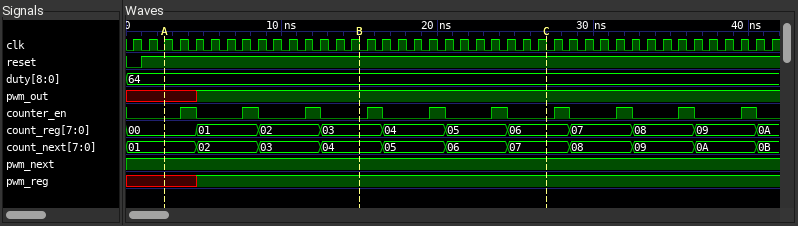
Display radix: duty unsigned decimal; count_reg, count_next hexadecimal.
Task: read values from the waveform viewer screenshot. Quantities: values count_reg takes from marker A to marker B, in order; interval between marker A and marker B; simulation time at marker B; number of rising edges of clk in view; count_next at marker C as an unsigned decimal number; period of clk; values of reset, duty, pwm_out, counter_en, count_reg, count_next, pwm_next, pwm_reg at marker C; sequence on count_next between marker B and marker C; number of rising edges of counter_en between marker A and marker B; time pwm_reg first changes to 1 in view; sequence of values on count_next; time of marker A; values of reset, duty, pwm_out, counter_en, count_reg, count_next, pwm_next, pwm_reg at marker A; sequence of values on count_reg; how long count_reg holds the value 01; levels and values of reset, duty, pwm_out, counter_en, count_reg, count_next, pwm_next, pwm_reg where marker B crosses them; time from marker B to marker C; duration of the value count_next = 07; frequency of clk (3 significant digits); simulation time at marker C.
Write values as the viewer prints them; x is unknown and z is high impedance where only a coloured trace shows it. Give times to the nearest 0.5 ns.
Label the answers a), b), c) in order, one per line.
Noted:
a) 00, 01, 02, 03
b) 12.5 ns
c) 15 ns
d) 42
e) 7
f) 1 ns
g) reset=1, duty=64, pwm_out=1, counter_en=0, count_reg=06, count_next=07, pwm_next=1, pwm_reg=1
h) 04, 05, 06, 07
i) 3
j) 4.5 ns
k) 01, 02, 03, 04, 05, 06, 07, 08, 09, 0A, 0B
l) 2.5 ns
m) reset=1, duty=64, pwm_out=x, counter_en=0, count_reg=00, count_next=01, pwm_next=1, pwm_reg=x
n) 00, 01, 02, 03, 04, 05, 06, 07, 08, 09, 0A
o) 4 ns
p) reset=1, duty=64, pwm_out=1, counter_en=0, count_reg=03, count_next=04, pwm_next=1, pwm_reg=1
q) 12 ns
r) 4 ns
s) 1.00 GHz
t) 27 ns
